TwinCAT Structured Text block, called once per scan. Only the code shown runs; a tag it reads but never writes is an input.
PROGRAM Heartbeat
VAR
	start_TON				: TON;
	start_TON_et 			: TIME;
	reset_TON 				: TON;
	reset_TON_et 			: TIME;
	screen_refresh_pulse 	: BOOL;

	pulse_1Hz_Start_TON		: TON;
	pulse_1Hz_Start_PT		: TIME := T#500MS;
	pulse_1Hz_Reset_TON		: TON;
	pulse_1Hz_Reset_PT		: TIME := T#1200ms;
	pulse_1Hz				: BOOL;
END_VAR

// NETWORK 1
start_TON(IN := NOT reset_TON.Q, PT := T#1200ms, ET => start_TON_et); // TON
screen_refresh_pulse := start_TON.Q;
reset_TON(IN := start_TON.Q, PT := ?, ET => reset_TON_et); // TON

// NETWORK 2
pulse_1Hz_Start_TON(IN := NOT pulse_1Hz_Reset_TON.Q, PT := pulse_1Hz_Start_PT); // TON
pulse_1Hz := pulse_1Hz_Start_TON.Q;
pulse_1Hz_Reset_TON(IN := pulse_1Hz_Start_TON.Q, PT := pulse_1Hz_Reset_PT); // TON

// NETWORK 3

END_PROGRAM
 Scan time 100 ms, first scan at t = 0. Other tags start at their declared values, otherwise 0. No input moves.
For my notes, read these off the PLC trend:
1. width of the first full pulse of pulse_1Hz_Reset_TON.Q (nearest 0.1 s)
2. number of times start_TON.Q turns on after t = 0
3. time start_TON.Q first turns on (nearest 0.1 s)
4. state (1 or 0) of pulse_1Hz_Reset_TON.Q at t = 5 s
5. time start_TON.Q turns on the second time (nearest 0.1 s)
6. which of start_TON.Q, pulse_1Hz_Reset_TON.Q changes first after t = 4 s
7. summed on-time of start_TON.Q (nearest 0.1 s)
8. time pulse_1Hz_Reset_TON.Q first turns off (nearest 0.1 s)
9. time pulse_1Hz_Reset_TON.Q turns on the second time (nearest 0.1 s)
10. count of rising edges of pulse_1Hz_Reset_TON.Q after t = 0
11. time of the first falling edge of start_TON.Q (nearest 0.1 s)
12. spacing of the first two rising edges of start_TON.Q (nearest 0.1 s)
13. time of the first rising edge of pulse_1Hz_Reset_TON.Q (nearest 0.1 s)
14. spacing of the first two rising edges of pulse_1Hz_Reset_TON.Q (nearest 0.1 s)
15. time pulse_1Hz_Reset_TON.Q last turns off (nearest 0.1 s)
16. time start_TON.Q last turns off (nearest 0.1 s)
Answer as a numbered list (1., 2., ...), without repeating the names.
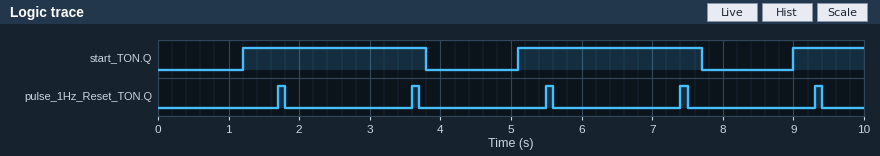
1. 0.1 s
2. 3
3. 1.2 s
4. 0
5. 5.1 s
6. start_TON.Q
7. 6.2 s
8. 1.8 s
9. 3.6 s
10. 5
11. 3.8 s
12. 3.9 s
13. 1.7 s
14. 1.9 s
15. 9.4 s
16. 7.7 s
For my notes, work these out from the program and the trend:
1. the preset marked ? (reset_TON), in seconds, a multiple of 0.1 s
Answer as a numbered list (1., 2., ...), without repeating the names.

1. 2.5 s
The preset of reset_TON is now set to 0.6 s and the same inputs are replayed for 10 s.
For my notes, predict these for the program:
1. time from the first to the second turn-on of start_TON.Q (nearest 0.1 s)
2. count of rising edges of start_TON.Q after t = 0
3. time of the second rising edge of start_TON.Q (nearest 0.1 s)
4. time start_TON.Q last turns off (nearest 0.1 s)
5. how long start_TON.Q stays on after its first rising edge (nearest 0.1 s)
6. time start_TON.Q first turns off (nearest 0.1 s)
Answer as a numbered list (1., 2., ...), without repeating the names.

1. 2.0 s
2. 5
3. 3.2 s
4. 9.9 s
5. 0.7 s
6. 1.9 s
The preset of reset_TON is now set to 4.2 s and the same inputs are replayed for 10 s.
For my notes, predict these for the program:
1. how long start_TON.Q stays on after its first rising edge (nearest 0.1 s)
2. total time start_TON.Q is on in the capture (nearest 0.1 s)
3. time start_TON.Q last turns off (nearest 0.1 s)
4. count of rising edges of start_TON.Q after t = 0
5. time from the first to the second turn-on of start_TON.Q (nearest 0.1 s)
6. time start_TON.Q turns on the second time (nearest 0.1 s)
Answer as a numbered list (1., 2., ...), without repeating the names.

1. 4.3 s
2. 7.5 s
3. 5.5 s
4. 2
5. 5.6 s
6. 6.8 s
